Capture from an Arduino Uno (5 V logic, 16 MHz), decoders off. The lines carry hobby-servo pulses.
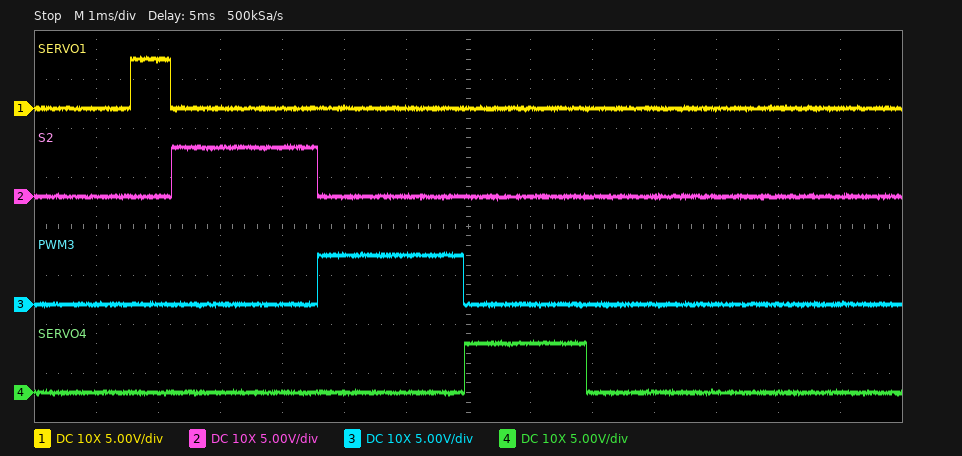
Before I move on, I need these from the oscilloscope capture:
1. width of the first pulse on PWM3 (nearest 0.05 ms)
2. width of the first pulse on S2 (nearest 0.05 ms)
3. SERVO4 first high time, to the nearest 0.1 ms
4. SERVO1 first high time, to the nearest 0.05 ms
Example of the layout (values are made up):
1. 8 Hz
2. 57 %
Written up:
1. 2.35 ms
2. 2.35 ms
3. 2.0 ms
4. 0.65 ms
